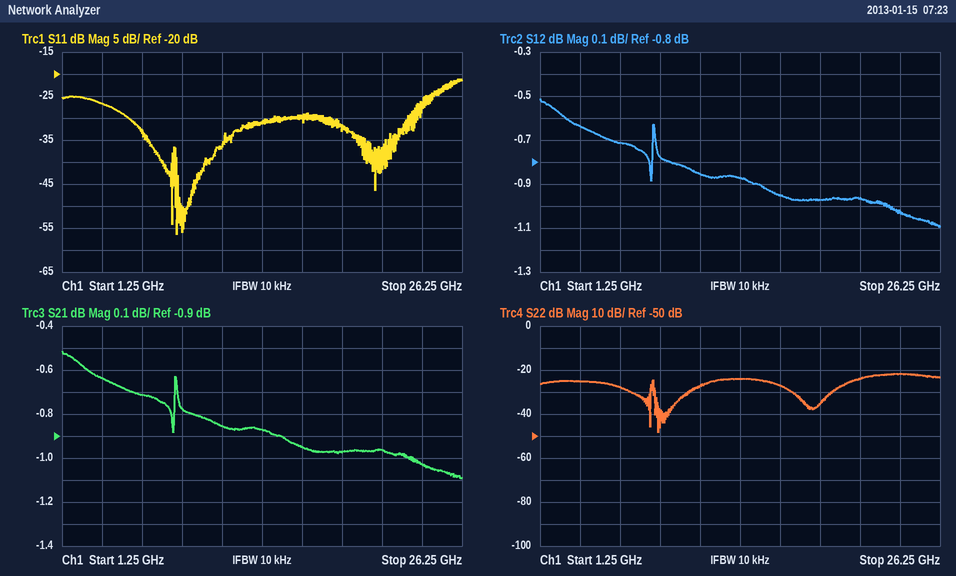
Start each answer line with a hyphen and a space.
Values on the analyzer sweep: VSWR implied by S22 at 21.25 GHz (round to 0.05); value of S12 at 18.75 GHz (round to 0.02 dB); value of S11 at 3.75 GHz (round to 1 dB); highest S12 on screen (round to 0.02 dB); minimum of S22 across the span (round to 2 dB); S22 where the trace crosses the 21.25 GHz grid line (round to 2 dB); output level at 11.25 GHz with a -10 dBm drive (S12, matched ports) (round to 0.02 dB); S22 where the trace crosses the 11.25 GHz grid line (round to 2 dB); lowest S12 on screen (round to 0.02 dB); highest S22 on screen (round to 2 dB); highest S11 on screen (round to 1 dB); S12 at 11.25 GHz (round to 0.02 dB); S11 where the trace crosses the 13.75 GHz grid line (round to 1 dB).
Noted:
- 1.15
- -0.98 dB
- -27 dB
- -0.52 dB
- -48 dB
- -24 dB
- -10.86 dBm
- -28 dB
- -1.10 dB
- -22 dB
- -21 dB
- -0.86 dB
- -31 dB
